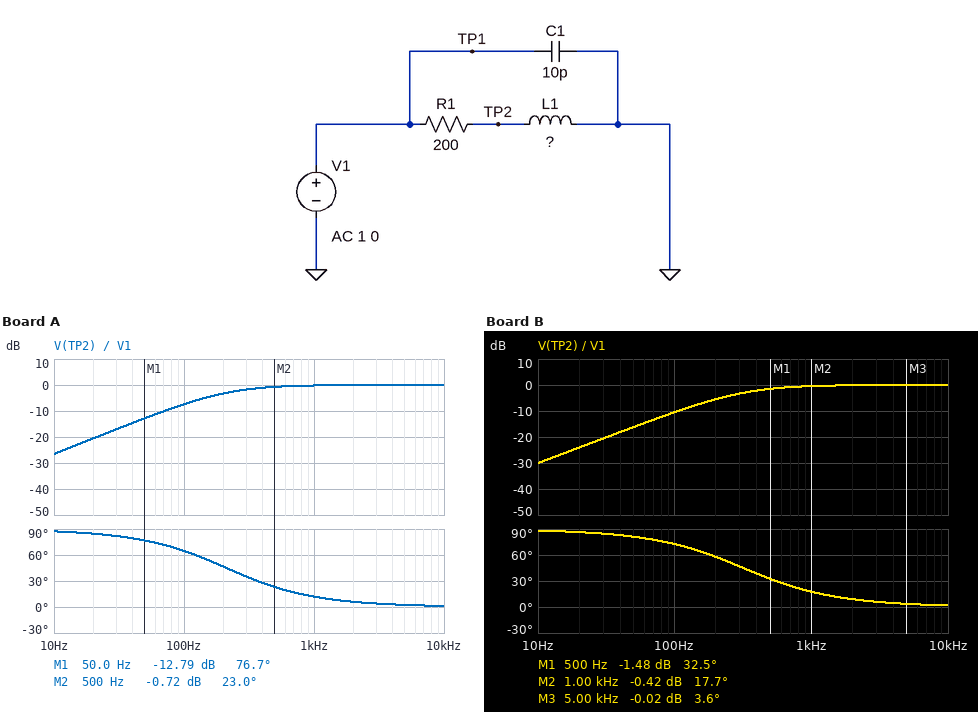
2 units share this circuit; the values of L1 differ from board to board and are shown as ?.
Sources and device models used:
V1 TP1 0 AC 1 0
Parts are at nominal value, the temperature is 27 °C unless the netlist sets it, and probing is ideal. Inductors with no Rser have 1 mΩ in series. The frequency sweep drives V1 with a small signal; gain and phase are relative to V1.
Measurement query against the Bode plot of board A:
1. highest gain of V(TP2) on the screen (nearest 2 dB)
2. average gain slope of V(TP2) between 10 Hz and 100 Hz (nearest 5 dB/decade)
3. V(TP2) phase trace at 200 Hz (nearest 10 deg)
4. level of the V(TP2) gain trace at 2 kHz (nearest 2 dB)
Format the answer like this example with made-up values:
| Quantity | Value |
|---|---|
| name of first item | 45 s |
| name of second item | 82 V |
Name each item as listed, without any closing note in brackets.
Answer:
| Quantity | Value |
|---|---|
| highest gain of V(TP2) on the screen | 0 dB |
| average gain slope of V(TP2) between 10 Hz and 100 Hz | 20 dB/decade |
| V(TP2) phase trace at 200 Hz | 50 deg |
| level of the V(TP2) gain trace at 2 kHz | 0 dB |
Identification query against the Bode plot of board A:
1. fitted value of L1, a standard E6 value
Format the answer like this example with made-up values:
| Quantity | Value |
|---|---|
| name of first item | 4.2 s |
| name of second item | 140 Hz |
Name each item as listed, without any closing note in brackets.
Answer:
| Quantity | Value |
|---|---|
| fitted value of L1, a standard E6 value | 150 mH |
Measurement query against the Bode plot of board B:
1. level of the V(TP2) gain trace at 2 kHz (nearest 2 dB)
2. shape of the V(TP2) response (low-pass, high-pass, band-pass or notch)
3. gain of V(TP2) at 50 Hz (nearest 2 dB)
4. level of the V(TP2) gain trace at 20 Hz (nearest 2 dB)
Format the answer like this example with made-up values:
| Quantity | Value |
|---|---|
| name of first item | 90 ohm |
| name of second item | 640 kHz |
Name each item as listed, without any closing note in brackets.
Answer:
| Quantity | Value |
|---|---|
| level of the V(TP2) gain trace at 2 kHz | 0 dB |
| shape of the V(TP2) response | high-pass |
| gain of V(TP2) at 50 Hz | -16 dB |
| level of the V(TP2) gain trace at 20 Hz | -24 dB |
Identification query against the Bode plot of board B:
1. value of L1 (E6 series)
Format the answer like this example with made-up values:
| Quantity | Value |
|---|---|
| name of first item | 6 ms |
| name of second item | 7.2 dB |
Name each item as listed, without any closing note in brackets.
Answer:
| Quantity | Value |
|---|---|
| value of L1 | 100 mH |
